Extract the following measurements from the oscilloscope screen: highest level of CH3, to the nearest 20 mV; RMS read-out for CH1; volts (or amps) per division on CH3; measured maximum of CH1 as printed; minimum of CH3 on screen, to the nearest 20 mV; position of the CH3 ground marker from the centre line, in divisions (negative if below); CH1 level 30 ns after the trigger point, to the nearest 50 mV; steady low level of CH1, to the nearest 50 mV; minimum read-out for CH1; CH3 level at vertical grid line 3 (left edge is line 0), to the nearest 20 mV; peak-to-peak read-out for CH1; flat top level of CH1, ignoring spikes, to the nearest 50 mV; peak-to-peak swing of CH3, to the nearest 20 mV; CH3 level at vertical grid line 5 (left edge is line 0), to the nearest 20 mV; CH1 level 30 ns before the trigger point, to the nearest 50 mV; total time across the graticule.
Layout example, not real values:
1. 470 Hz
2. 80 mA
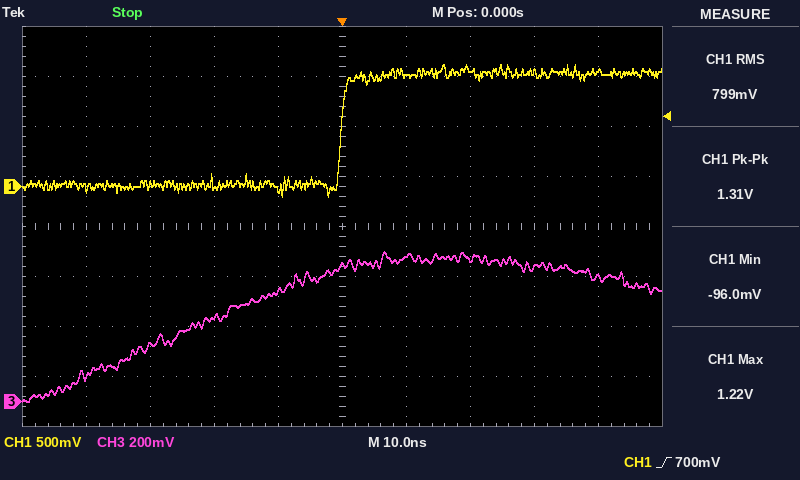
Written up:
1. 600 mV
2. 799 mV
3. 200 mV
4. 1.22 V
5. 0 mV
6. -3.5 div
7. 1.15 V
8. 0 mV
9. -96.0 mV
10. 340 mV
11. 1.31 V
12. 1.15 V
13. 600 mV
14. 540 mV
15. 0 mV
16. 100 ns
